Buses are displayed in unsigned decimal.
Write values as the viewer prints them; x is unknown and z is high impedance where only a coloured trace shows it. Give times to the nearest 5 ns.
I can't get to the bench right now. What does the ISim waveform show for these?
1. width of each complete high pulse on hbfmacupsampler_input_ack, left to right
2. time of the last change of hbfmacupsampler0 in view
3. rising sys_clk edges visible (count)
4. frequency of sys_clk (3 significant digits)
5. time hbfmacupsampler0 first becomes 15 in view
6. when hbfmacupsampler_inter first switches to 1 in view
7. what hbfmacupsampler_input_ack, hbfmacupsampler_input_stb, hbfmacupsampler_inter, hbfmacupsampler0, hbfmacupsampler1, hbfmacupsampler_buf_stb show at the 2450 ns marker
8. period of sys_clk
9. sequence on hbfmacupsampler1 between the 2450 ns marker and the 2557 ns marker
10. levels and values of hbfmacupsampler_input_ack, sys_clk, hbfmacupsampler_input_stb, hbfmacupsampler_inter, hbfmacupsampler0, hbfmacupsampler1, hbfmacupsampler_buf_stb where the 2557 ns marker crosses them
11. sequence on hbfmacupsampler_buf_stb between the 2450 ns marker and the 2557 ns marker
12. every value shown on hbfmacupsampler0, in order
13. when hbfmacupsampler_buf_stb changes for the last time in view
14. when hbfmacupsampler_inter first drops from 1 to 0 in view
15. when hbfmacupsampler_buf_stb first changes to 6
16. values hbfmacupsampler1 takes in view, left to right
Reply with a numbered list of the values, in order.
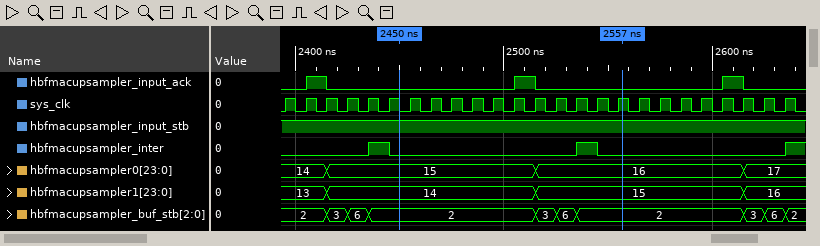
1. 10 ns, 10 ns, 10 ns
2. 2615 ns
3. 25
4. 100 MHz
5. 2415 ns
6. 2435 ns
7. hbfmacupsampler_input_ack=0, hbfmacupsampler_input_stb=1, hbfmacupsampler_inter=0, hbfmacupsampler0=15, hbfmacupsampler1=14, hbfmacupsampler_buf_stb=2
8. 10 ns
9. 14, 15
10. hbfmacupsampler_input_ack=0, sys_clk=1, hbfmacupsampler_input_stb=1, hbfmacupsampler_inter=0, hbfmacupsampler0=16, hbfmacupsampler1=15, hbfmacupsampler_buf_stb=2
11. 2, 3, 6, 2
12. 14, 15, 16, 17
13. 2635 ns
14. 2445 ns
15. 2425 ns
16. 13, 14, 15, 16
